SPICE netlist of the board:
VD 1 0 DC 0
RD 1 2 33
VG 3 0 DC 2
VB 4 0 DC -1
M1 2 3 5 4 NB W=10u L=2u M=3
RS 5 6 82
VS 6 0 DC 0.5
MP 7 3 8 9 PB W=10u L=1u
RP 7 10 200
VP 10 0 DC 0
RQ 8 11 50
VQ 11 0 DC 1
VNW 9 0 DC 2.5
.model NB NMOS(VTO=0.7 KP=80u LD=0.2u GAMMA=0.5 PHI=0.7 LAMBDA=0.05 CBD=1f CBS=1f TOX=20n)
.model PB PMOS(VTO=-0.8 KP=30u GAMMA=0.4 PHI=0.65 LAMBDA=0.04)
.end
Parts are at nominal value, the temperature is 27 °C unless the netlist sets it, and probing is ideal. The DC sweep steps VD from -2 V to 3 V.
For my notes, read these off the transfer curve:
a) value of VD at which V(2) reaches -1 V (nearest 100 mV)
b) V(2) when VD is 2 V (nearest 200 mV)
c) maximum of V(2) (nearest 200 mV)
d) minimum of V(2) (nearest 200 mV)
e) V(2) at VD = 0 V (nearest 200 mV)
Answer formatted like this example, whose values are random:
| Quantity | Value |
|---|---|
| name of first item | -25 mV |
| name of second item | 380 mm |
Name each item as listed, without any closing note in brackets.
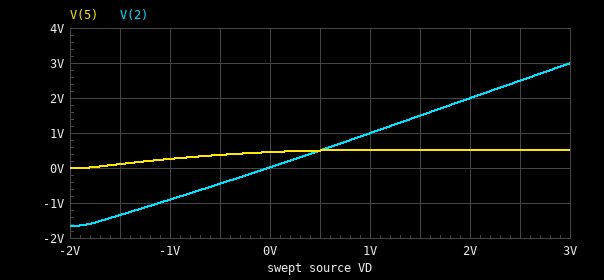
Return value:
| Quantity | Value |
|---|---|
| value of VD at which V(2) reaches -1 V | -1.1 V |
| V(2) when VD is 2 V | 2.0 V |
| maximum of V(2) | 3.0 V |
| minimum of V(2) | -1.6 V |
| V(2) at VD = 0 V | 0 V |
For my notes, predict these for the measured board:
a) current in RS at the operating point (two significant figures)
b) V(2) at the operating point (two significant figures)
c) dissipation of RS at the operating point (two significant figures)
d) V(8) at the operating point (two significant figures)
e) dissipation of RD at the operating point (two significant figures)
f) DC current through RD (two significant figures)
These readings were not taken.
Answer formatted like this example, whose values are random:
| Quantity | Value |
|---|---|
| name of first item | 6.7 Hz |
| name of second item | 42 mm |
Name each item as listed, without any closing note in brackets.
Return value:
| Quantity | Value |
|---|---|
| current in RS at the operating point | 550 µA |
| V(2) at the operating point | 18 mV |
| dissipation of RS at the operating point | 25 µW |
| V(8) at the operating point | 1.0 V |
| dissipation of RD at the operating point | 10 µW |
| DC current through RD | 550 µA |
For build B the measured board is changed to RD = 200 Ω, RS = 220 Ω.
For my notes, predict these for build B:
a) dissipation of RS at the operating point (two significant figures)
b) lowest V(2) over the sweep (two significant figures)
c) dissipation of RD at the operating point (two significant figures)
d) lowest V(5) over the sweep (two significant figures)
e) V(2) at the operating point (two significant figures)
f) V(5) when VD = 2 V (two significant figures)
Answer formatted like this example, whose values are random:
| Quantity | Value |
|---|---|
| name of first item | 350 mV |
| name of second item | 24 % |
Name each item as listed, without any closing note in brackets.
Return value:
| Quantity | Value |
|---|---|
| dissipation of RS at the operating point | 36 µW |
| lowest V(2) over the sweep | -1.3 V |
| dissipation of RD at the operating point | 33 µW |
| lowest V(5) over the sweep | -270 mV |
| V(2) at the operating point | 81 mV |
| V(5) when VD = 2 V | 530 mV |
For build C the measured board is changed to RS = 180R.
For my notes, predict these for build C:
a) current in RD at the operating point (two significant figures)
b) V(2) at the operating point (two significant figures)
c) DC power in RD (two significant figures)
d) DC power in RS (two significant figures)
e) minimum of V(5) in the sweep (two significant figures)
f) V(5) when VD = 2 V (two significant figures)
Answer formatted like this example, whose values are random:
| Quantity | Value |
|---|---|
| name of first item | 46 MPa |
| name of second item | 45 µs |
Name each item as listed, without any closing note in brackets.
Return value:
| Quantity | Value |
|---|---|
| current in RD at the operating point | 510 µA |
| V(2) at the operating point | 17 mV |
| DC power in RD | 8.6 µW |
| DC power in RS | 47 µW |
| minimum of V(5) in the sweep | -410 mV |
| V(5) when VD = 2 V | 530 mV |
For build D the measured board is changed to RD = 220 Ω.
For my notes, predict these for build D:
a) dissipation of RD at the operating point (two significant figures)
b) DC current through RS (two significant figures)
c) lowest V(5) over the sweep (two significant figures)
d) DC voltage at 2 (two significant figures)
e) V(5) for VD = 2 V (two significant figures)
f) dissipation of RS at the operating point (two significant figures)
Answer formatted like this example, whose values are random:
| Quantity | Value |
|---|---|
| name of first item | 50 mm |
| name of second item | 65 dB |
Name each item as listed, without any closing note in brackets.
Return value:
| Quantity | Value |
|---|---|
| dissipation of RD at the operating point | 41 µW |
| DC current through RS | 430 µA |
| lowest V(5) over the sweep | 180 mV |
| DC voltage at 2 | 95 mV |
| V(5) for VD = 2 V | 510 mV |
| dissipation of RS at the operating point | 15 µW |
